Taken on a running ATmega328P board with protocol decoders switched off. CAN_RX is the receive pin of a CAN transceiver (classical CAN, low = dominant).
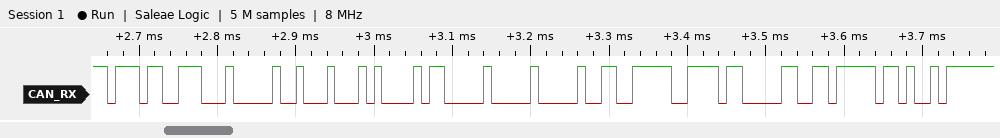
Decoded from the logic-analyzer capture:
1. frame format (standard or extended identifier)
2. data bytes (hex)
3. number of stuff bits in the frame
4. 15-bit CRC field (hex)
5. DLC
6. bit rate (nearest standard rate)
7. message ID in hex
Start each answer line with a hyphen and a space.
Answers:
- standard
- 08 8A 16 00 00 CF BD 82
- 7
- 0x37F4
- 8
- 100 kbit/s
- 0x767
